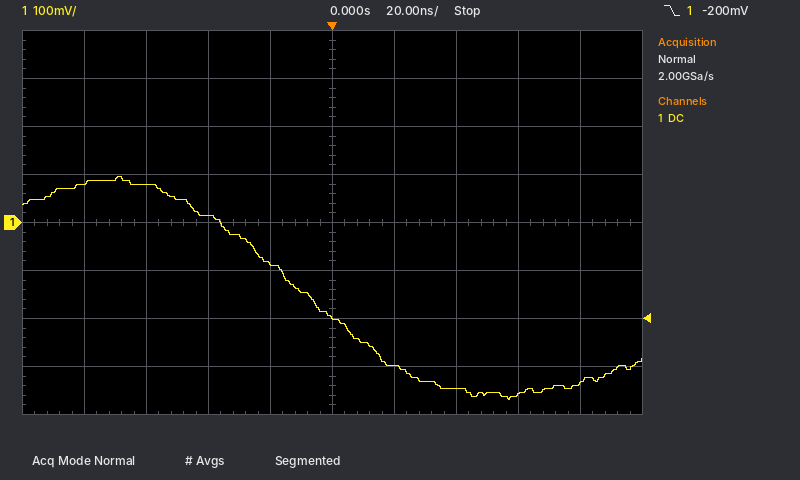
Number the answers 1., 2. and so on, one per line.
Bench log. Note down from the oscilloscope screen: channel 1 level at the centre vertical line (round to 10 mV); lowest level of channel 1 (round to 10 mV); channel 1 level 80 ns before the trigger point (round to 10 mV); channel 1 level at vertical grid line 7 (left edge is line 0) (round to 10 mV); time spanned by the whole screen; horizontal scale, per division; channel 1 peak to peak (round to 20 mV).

1. -200 mV
2. -370 mV
3. 80 mV
4. -350 mV
5. 200 ns
6. 20 ns
7. 460 mV
